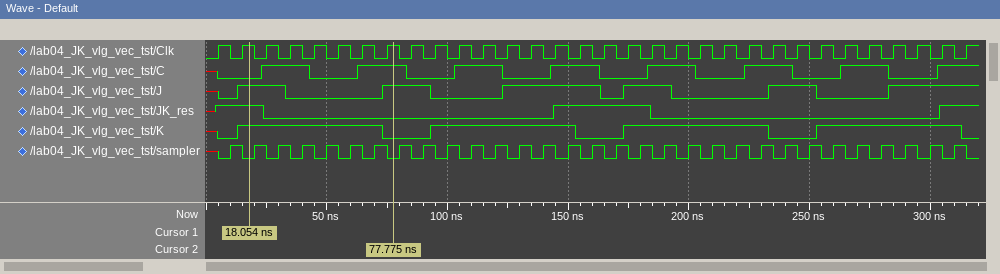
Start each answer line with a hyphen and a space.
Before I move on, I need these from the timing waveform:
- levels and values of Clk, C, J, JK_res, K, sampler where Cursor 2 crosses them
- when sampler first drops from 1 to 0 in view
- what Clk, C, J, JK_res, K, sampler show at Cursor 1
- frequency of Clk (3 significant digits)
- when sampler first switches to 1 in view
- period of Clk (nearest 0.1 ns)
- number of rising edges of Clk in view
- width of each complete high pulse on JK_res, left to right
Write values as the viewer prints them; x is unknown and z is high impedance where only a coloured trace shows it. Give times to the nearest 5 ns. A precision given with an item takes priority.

- Clk=1, C=1, J=1, JK_res=0, K=0, sampler=0
- 15 ns
- Clk=1, C=0, J=1, JK_res=1, K=1, sampler=0
- 100 MHz
- 10 ns
- 10 ns
- 32
- 40 ns
